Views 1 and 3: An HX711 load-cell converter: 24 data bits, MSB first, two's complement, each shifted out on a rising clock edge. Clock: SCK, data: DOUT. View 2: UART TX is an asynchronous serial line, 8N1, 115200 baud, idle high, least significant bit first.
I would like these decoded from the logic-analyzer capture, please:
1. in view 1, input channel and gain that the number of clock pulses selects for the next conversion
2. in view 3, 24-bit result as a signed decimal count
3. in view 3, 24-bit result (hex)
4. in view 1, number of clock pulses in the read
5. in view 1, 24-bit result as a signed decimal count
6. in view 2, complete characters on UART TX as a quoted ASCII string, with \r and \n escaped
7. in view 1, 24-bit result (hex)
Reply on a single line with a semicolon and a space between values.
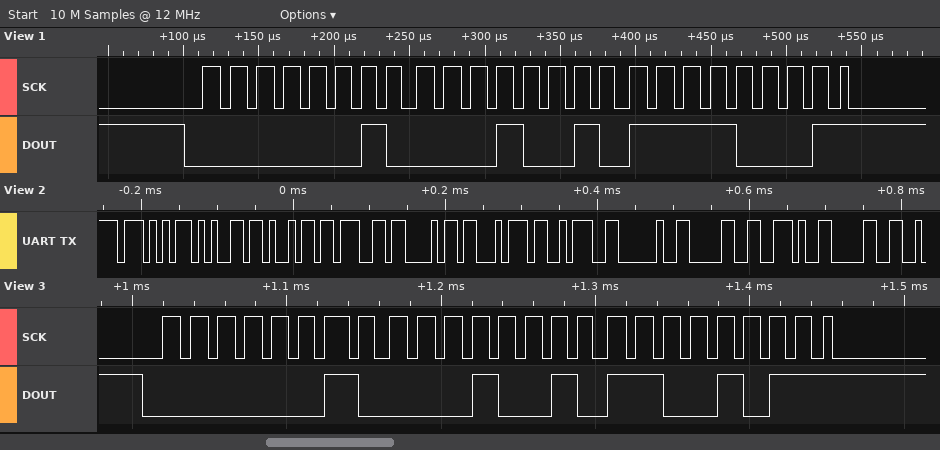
channel A, gain 128; 135883; 0x0212CB; 25; 135921; "Weight: 0.0"; 0x0212F1
